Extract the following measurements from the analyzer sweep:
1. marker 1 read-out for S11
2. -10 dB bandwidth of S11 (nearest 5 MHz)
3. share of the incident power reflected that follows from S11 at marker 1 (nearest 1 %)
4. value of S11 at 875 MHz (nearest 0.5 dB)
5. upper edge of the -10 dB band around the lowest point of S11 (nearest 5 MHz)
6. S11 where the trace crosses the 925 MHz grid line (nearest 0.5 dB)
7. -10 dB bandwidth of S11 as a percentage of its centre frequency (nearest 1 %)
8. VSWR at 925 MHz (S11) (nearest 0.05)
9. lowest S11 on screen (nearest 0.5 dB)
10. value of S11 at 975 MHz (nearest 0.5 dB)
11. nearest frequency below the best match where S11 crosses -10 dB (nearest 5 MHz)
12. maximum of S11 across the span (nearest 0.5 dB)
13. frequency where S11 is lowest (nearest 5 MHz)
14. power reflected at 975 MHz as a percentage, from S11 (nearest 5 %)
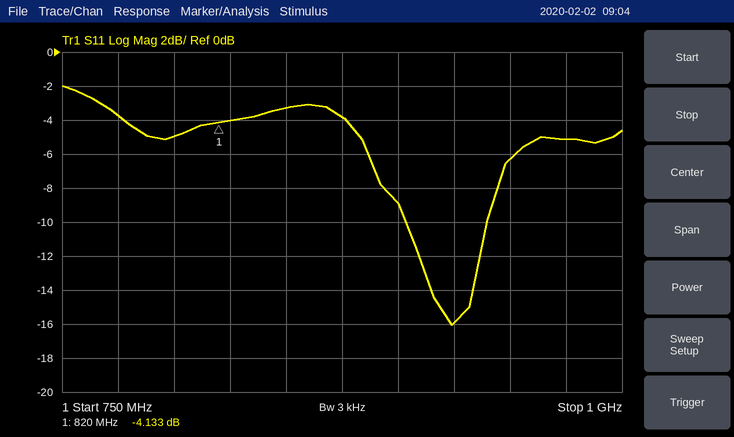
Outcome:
-4.133 dB
35 MHz
39 %
-4.0 dB
940 MHz
-16.0 dB
4 %
1.40
-16.0 dB
-5.0 dB
905 MHz
-2.0 dB
925 MHz
30 %
